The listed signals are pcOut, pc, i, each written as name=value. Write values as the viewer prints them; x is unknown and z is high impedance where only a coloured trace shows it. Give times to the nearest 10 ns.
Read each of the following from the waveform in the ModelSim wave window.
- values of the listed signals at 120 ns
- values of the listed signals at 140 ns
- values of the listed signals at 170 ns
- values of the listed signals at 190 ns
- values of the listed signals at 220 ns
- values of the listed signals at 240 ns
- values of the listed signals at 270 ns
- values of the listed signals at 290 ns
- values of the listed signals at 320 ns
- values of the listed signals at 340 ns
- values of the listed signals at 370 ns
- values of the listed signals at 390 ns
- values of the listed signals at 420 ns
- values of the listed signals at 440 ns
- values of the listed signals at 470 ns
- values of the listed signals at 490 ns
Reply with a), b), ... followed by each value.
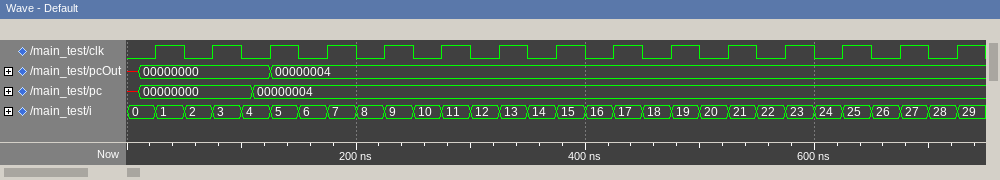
a) pcOut=00000000, pc=00000004, i=4
b) pcOut=00000004, pc=00000004, i=5
c) pcOut=00000004, pc=00000004, i=6
d) pcOut=00000004, pc=00000004, i=7
e) pcOut=00000004, pc=00000004, i=8
f) pcOut=00000004, pc=00000004, i=9
g) pcOut=00000004, pc=00000004, i=10
h) pcOut=00000004, pc=00000004, i=11
i) pcOut=00000004, pc=00000004, i=12
j) pcOut=00000004, pc=00000004, i=13
k) pcOut=00000004, pc=00000004, i=14
l) pcOut=00000004, pc=00000004, i=15
m) pcOut=00000004, pc=00000004, i=16
n) pcOut=00000004, pc=00000004, i=17
o) pcOut=00000004, pc=00000004, i=18
p) pcOut=00000004, pc=00000004, i=19
